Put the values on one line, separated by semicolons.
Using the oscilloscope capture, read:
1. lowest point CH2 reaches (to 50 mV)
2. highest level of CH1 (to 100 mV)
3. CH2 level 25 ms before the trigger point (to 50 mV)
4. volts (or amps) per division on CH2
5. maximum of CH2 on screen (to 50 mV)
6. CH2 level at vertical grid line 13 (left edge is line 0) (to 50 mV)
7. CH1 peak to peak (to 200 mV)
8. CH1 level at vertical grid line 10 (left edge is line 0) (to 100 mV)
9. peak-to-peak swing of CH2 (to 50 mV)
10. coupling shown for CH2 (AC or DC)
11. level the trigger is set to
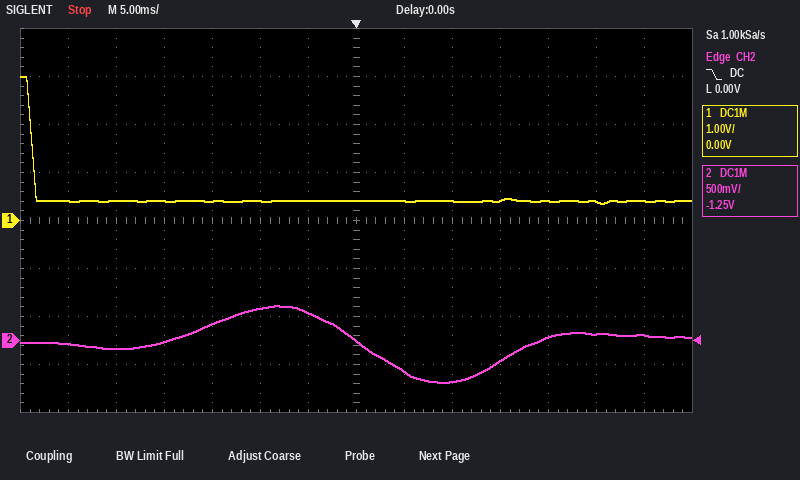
-450 mV; 3.0 V; -100 mV; 500 mV; 350 mV; 50 mV; 2.6 V; 400 mV; 800 mV; DC; 0.00 V
